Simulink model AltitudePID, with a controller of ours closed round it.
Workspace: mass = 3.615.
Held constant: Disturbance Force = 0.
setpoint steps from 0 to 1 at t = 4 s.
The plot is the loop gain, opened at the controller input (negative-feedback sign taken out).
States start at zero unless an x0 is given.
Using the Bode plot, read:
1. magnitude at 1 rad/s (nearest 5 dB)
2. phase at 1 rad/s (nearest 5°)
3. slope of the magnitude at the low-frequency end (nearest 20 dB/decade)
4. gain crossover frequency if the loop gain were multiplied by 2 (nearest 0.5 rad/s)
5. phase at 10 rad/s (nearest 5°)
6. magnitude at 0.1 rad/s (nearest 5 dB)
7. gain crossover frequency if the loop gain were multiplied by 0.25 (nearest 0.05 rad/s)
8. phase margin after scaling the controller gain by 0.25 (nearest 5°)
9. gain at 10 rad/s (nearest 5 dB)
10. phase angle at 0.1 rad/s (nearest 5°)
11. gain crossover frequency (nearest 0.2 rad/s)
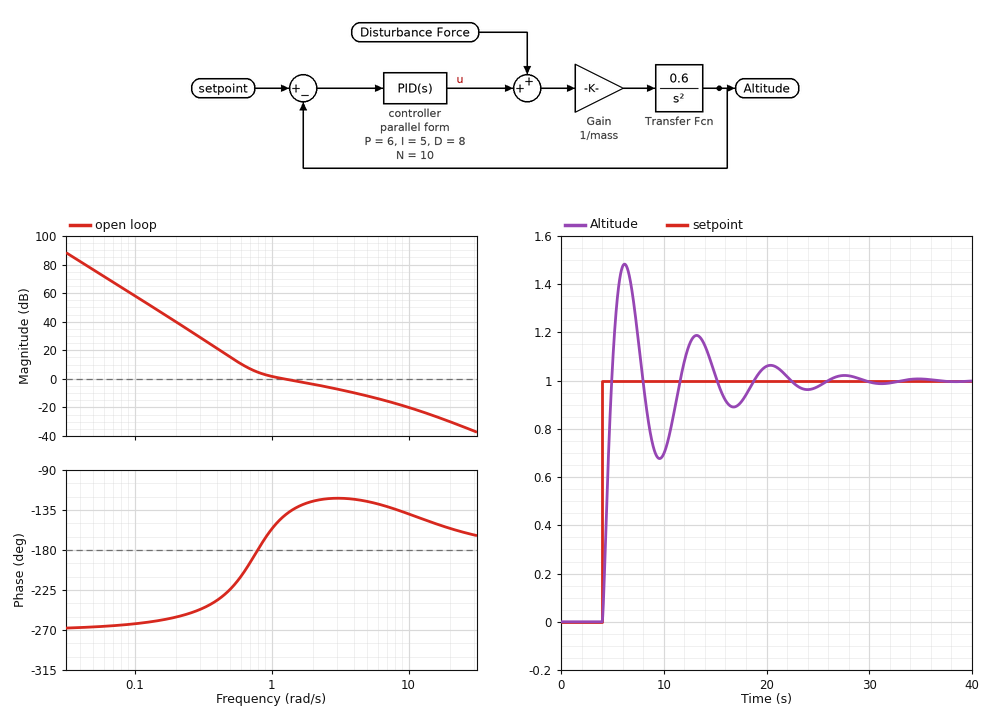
0 dB
-155°
-60 dB/decade
2.5 rad/s
-140°
60 dB
0.55 rad/s
-35°
-20 dB
-265°
1.2 rad/s
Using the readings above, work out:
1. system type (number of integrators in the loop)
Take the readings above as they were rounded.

3
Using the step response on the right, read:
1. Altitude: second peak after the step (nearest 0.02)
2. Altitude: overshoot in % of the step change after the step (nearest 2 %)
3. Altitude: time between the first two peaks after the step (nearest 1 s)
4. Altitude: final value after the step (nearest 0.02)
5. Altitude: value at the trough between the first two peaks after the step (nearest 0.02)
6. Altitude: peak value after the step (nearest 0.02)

1.18
48 %
7 s
1.00
0.68
1.48
